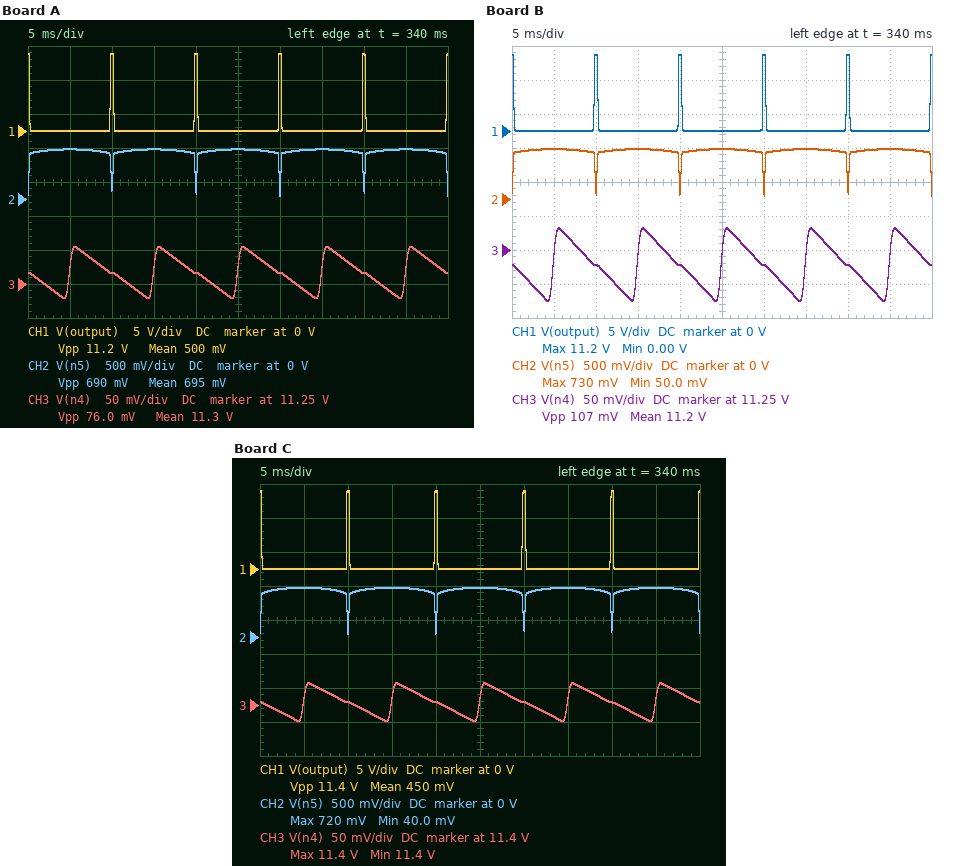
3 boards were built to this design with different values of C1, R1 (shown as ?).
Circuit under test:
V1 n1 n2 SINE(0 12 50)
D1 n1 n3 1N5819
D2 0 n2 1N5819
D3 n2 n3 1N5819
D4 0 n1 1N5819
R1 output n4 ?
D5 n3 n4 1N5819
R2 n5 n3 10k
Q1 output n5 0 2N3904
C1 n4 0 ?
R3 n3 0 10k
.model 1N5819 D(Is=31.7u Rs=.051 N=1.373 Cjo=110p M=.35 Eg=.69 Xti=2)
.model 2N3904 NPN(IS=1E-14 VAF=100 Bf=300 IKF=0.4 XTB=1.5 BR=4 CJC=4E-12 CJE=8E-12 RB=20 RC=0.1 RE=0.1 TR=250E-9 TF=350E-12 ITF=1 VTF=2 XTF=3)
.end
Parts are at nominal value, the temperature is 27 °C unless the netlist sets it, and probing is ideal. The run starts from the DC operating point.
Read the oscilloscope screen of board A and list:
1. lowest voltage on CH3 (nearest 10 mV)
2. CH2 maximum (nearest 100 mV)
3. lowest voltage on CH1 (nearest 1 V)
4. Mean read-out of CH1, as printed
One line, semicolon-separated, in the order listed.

11.23 V; 700 mV; 0 V; 500 mV
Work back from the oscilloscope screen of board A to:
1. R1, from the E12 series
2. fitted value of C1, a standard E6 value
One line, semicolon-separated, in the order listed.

5.6 kΩ; 220 µF
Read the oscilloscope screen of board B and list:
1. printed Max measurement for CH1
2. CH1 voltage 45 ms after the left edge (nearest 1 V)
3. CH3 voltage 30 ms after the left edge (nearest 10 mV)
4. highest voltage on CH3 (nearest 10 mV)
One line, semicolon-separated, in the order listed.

11.2 V; 0 V; 11.23 V; 11.28 V
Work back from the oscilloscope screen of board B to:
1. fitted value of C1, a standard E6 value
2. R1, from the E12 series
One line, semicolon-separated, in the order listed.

220 µF; 3.9 kΩ
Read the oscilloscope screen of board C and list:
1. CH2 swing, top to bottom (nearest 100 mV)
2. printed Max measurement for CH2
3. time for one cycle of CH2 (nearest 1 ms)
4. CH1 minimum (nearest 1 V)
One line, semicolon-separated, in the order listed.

700 mV; 720 mV; 10 ms; 0 V
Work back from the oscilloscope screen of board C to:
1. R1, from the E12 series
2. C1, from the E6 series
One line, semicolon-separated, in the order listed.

27 kΩ; 68 µF
